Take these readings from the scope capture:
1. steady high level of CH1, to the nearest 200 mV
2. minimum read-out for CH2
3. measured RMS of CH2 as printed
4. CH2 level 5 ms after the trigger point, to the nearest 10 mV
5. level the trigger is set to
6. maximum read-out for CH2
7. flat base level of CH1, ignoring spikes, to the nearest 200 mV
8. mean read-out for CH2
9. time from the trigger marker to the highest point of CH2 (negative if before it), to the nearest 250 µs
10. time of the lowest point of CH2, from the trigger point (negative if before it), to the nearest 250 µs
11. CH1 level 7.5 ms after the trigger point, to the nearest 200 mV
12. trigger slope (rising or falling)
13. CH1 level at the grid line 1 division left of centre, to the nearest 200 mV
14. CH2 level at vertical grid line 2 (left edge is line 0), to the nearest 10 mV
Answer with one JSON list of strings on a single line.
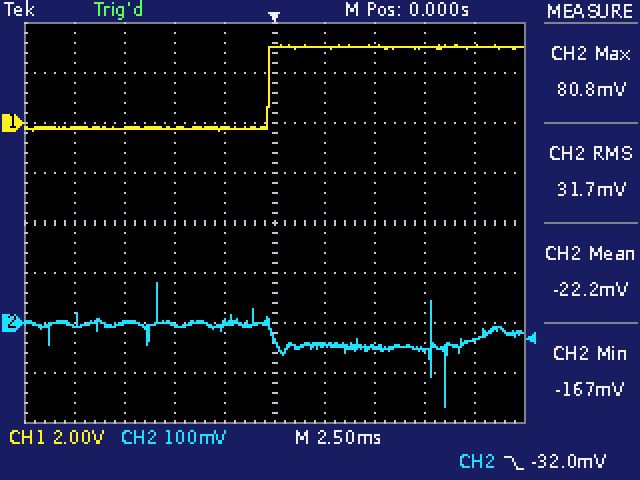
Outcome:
["3.0 V", "-167 mV", "31.7 mV", "-50 mV", "-32.0 mV", "80.8 mV", "-200 mV", "-22.2 mV", "-5.75 ms", "+8.50 ms", "3.0 V", "falling", "-200 mV", "0 mV"]
